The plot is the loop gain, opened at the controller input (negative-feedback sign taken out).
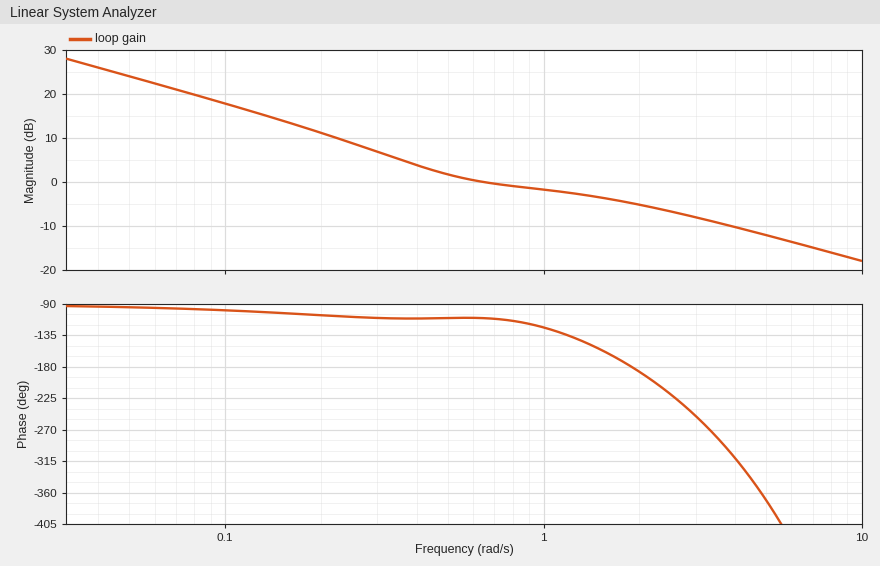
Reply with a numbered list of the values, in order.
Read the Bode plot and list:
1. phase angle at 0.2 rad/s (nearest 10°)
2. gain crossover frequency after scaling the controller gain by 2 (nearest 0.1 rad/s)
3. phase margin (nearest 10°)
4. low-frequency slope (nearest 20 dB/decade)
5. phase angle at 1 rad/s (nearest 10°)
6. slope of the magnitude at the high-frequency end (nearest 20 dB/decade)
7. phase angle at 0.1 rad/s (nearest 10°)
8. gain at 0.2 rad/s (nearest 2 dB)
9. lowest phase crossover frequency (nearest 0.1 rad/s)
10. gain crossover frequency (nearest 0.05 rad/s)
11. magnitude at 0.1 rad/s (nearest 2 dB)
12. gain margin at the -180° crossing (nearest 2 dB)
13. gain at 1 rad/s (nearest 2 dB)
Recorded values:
1. -110°
2. 2.3 rad/s
3. 70°
4. -20 dB/decade
5. -120°
6. -20 dB/decade
7. -100°
8. 12 dB
9. 1.9 rad/s
10. 0.65 rad/s
11. 18 dB
12. 4 dB
13. -2 dB
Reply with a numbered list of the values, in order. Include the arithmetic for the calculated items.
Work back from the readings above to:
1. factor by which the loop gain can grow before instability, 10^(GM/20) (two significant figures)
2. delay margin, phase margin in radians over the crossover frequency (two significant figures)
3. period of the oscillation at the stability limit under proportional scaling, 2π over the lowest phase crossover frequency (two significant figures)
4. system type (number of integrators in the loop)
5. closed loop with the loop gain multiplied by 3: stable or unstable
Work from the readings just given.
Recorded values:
1. 10^(4 / 20) = 1.6
2. 70 × π / 180 / 0.65 = 1.9 s
3. 2π / 1.9 = 3.3 s
4. 1
5. unstable
